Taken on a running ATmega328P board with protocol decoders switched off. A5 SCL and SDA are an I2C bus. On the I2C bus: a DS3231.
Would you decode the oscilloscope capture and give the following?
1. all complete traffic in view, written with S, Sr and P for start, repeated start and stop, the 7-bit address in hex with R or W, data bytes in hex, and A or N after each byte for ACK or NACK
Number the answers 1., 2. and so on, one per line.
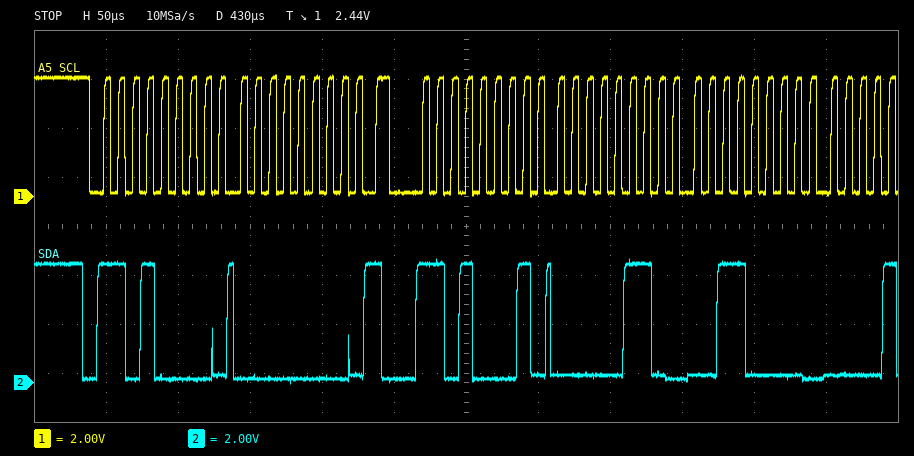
1. S 68W A 00 A Sr 68R A 06 A 30 A
